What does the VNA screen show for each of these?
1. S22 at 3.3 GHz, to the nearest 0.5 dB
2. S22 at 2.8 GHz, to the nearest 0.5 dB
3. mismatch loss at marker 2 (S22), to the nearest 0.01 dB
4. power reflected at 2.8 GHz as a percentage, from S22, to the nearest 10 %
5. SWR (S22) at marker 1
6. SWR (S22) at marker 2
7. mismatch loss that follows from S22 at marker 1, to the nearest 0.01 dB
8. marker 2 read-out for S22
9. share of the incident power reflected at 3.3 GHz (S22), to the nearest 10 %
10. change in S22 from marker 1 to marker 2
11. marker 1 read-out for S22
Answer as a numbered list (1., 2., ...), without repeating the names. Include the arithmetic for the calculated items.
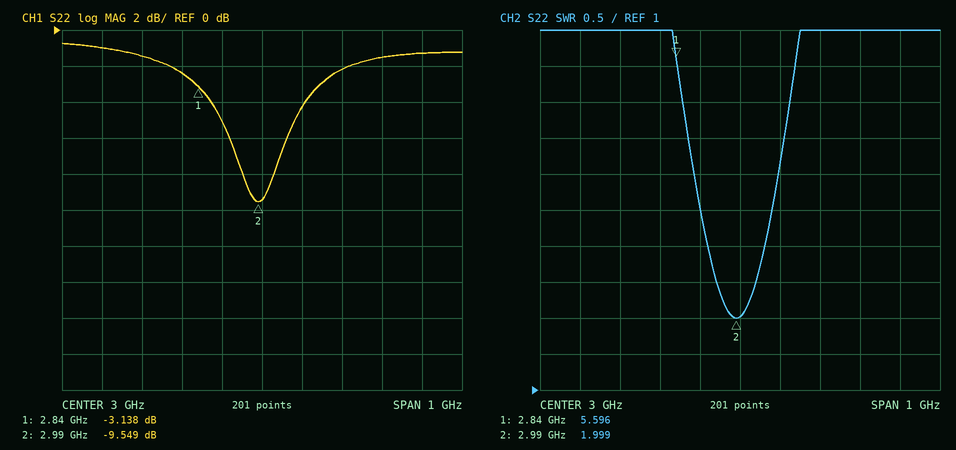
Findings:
1. -1.5 dB
2. -2.5 dB
3. −10 log10(1 − 10^(-9.549/10)) ≈ 0.51 dB
4. 10^(-2.5/10) ≈ 56.2 %, so 60 % to the nearest 10 %
5. 5.596
6. 1.999
7. −10 log10(1 − 10^(-3.138/10)) ≈ 2.89 dB
8. -9.549 dB
9. 10^(-1.5/10) ≈ 70.8 %, so 70 % to the nearest 10 %
10. -9.549 − (-3.138) = -6.411 dB
11. -3.138 dB
